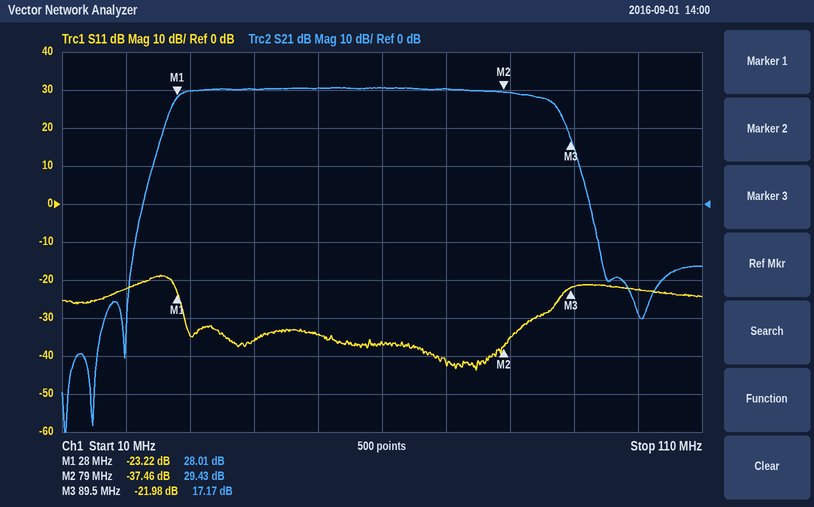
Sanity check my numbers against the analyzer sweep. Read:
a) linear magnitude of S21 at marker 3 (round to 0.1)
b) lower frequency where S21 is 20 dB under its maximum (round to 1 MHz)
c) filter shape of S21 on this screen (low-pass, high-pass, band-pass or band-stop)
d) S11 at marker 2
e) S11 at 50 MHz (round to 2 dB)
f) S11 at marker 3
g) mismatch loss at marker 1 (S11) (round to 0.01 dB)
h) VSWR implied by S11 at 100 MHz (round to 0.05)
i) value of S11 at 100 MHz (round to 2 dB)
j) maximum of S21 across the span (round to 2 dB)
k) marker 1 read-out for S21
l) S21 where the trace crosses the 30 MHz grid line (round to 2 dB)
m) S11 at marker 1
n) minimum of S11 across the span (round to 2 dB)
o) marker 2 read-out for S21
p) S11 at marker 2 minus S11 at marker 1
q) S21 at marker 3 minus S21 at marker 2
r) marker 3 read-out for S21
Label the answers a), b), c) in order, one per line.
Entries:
a) 7.2
b) 24 MHz
c) band-pass
d) -37.46 dB
e) -34 dB
f) -21.98 dB
g) 0.02 dB
h) 1.15
i) -22 dB
j) 30 dB
k) 28.01 dB
l) 30 dB
m) -23.22 dB
n) -44 dB
o) 29.43 dB
p) -14.24 dB
q) -12.26 dB
r) 17.17 dB
